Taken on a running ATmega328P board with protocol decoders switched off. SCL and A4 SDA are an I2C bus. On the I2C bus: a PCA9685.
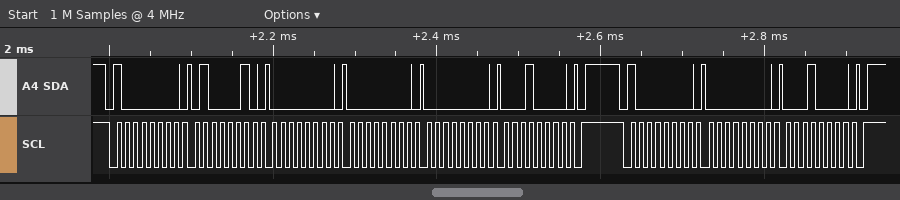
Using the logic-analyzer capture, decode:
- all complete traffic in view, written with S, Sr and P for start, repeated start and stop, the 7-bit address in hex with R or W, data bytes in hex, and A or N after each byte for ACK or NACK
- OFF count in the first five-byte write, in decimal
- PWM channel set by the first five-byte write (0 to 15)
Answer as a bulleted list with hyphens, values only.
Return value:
- S 40W A 42 A 00 A 00 A 00 A 10 A P S 40W A 00 A 10 A P
- 4096
- 15
